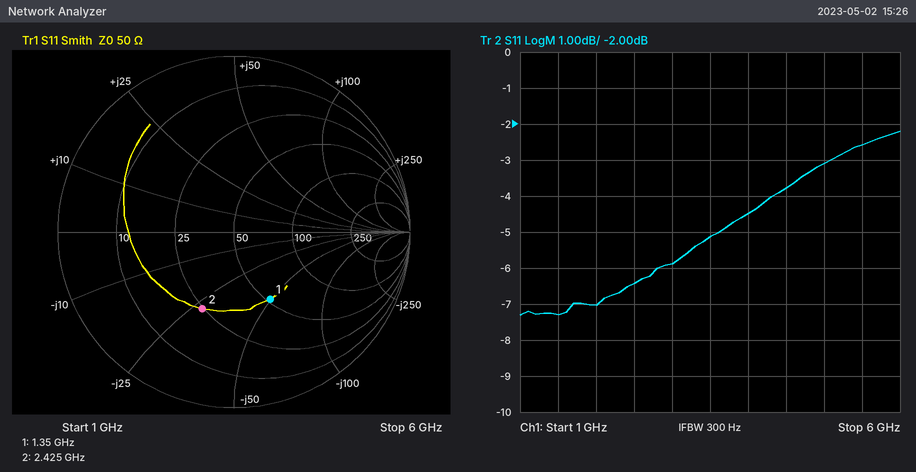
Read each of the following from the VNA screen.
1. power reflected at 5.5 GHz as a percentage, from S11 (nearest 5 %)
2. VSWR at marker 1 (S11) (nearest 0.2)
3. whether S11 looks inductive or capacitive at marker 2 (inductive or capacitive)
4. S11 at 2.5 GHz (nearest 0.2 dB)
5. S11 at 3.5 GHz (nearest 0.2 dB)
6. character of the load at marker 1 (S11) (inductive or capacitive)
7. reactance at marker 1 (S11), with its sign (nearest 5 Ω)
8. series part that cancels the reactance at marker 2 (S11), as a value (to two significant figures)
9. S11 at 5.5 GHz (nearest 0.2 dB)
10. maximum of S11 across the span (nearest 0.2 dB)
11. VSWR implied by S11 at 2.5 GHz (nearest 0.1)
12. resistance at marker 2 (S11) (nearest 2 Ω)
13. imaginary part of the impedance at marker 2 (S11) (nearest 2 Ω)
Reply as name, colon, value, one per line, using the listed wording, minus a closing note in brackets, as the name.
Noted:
power reflected at 5.5 GHz as a percentage, from S11: 55 %
VSWR at marker 1 (S11): 2.6
whether S11 looks inductive or capacitive at marker 2: capacitive
S11 at 2.5 GHz: -6.4 dB
S11 at 3.5 GHz: -5.2 dB
character of the load at marker 1 (S11): capacitive
reactance at marker 1 (S11), with its sign: -50 Ω
series part that cancels the reactance at marker 2 (S11), as a value: 1.8 nH
S11 at 5.5 GHz: -2.6 dB
maximum of S11 across the span: -2.2 dB
VSWR implied by S11 at 2.5 GHz: 2.8
resistance at marker 2 (S11): 24 Ω
imaginary part of the impedance at marker 2 (S11): -28 Ω
